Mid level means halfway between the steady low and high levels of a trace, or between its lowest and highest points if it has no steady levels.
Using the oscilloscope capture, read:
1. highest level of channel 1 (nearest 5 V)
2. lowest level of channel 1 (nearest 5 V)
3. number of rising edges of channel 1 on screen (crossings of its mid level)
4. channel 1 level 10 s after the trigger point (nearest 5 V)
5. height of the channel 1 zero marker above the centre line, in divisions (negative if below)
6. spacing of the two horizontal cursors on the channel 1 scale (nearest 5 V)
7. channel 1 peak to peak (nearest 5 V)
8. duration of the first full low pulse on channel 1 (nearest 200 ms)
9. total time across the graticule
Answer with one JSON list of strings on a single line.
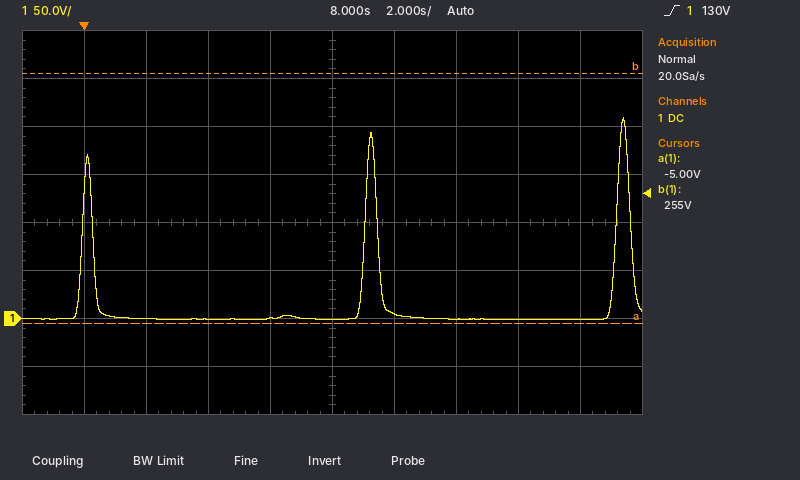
["210 V", "0 V", "3", "5 V", "-2.0 div", "260 V", "210 V", "8.8 s", "20 s"]
